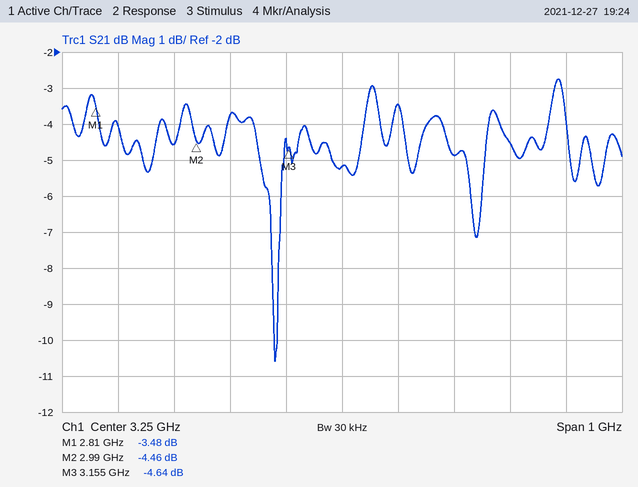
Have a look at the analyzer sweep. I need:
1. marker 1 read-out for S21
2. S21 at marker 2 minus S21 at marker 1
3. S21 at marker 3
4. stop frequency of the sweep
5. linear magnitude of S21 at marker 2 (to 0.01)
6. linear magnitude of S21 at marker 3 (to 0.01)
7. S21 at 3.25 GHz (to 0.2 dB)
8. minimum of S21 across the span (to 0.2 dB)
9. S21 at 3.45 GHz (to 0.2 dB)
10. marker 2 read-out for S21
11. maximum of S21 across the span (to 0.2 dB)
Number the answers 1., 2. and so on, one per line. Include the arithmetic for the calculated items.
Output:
1. -3.48 dB
2. -4.46 − (-3.48) = -0.98 dB
3. -4.64 dB
4. 3.75 GHz
5. 10^(-4.46/20) ≈ 0.60
6. 10^(-4.64/20) ≈ 0.59
7. -5.2 dB
8. -10.6 dB
9. -4.8 dB
10. -4.46 dB
11. -2.8 dB
